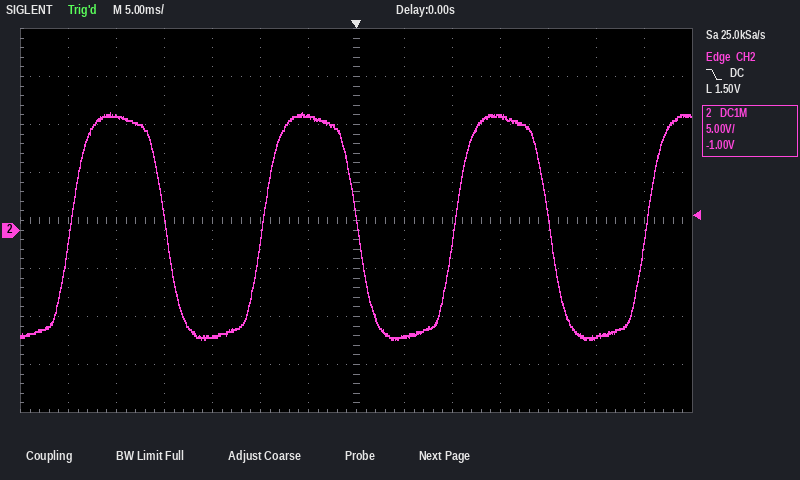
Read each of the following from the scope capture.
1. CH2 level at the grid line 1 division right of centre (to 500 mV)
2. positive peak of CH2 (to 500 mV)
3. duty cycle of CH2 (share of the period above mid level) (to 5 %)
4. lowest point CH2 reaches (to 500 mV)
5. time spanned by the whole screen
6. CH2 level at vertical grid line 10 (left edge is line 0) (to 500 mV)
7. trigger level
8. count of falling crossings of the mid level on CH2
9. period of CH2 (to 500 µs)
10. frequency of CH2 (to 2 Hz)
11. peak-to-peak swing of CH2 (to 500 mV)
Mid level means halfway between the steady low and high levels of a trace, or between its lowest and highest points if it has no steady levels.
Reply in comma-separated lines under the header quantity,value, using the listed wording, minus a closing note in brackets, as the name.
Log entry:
quantity,value
CH2 level at the grid line 1 division right of centre,-11.0 V
positive peak of CH2,12.0 V
duty cycle of CH2 (share of the period above mid level),50 %
lowest point CH2 reaches,-11.5 V
time spanned by the whole screen,70 ms
CH2 level at vertical grid line 10 (left edge is line 0),12.0 V
trigger level,1.50 V
count of falling crossings of the mid level on CH2,3
period of CH2,20.0 ms
frequency of CH2,50 Hz
peak-to-peak swing of CH2,23.5 V
